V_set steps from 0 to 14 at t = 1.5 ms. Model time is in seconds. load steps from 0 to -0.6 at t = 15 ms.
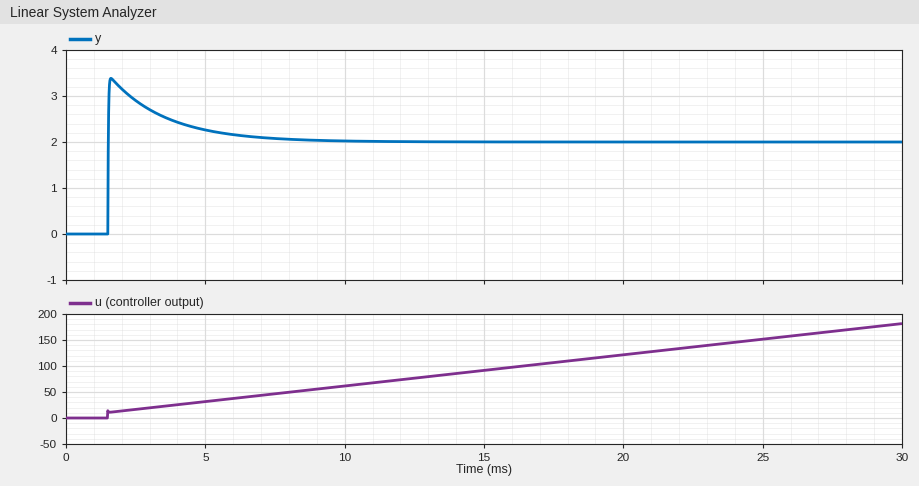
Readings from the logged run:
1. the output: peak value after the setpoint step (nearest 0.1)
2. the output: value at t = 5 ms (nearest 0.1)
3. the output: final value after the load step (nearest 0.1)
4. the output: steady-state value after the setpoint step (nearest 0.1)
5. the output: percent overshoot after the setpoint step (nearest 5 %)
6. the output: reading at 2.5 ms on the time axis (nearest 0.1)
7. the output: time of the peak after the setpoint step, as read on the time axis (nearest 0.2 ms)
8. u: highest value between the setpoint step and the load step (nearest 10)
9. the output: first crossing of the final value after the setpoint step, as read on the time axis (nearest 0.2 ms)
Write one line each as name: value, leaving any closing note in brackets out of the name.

the output: peak value after the setpoint step: 3.4
the output: value at t = 5 ms: 2.3
the output: final value after the load step: 2.0
the output: steady-state value after the setpoint step: 2.0
the output: percent overshoot after the setpoint step: 70 %
the output: reading at 2.5 ms on the time axis: 2.9
the output: time of the peak after the setpoint step, as read on the time axis: 1.6 ms
u: highest value between the setpoint step and the load step: 90
the output: first crossing of the final value after the setpoint step, as read on the time axis: 1.6 ms
